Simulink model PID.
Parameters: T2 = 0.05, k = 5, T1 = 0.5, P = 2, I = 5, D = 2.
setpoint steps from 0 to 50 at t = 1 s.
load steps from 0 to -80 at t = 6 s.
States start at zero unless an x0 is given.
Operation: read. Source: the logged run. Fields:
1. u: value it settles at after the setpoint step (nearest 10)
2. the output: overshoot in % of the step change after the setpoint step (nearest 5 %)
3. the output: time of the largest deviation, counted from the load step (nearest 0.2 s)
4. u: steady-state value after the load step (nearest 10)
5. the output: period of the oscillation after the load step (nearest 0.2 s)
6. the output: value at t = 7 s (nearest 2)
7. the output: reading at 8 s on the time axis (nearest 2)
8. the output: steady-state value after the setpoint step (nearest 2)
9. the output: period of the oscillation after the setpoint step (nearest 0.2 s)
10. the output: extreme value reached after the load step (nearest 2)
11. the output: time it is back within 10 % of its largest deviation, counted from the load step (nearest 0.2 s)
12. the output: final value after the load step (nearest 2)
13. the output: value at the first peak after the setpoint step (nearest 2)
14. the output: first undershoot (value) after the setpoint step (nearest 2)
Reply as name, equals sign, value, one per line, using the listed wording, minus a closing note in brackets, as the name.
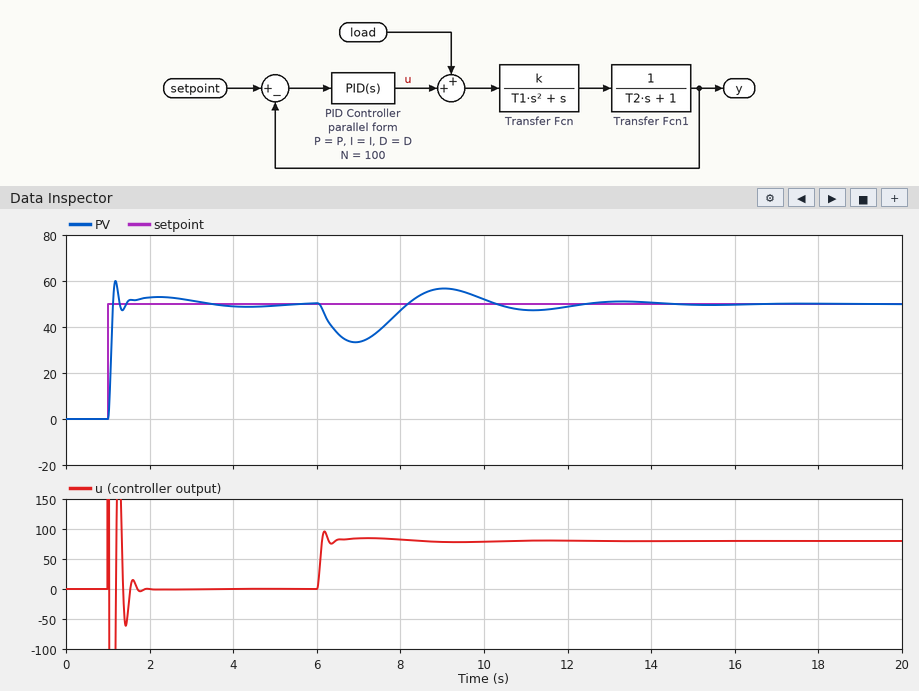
u: value it settles at after the setpoint step = 0
the output: overshoot in % of the step change after the setpoint step = 20 %
the output: time of the largest deviation, counted from the load step = 1.0 s
u: steady-state value after the load step = 80
the output: period of the oscillation after the load step = 4.2 s
the output: value at t = 7 s = 34
the output: reading at 8 s on the time axis = 48
the output: steady-state value after the setpoint step = 50
the output: period of the oscillation after the setpoint step = 1.0 s
the output: extreme value reached after the load step = 34
the output: time it is back within 10 % of its largest deviation, counted from the load step = 5.8 s
the output: final value after the load step = 50
the output: value at the first peak after the setpoint step = 60
the output: first undershoot (value) after the setpoint step = 48
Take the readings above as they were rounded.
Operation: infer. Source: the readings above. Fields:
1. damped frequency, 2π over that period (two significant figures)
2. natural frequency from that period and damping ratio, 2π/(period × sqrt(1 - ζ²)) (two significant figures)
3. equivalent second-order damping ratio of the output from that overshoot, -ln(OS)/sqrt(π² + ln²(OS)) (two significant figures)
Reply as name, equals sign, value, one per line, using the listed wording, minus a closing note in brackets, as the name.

damped frequency, 2π over that period = 6.3 rad/s
natural frequency from that period and damping ratio, 2π/(period × sqrt(1 - ζ²)) = 7.1 rad/s
equivalent second-order damping ratio of the output from that overshoot, -ln(OS)/sqrt(π² + ln²(OS)) = 0.46
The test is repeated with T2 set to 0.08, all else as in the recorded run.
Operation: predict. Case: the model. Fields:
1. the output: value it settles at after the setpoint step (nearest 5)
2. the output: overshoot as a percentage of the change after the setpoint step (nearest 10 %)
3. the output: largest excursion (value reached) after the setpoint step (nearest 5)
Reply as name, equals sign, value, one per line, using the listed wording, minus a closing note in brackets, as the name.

the output: value it settles at after the setpoint step = 50
the output: overshoot as a percentage of the change after the setpoint step = 30 %
the output: largest excursion (value reached) after the setpoint step = 65
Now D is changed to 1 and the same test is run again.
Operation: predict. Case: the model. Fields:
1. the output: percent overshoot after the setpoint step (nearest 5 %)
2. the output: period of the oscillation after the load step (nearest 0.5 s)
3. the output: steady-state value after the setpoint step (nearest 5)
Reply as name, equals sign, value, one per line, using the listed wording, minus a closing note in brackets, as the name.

the output: percent overshoot after the setpoint step = 15 %
the output: period of the oscillation after the load step = 3.0 s
the output: steady-state value after the setpoint step = 50
